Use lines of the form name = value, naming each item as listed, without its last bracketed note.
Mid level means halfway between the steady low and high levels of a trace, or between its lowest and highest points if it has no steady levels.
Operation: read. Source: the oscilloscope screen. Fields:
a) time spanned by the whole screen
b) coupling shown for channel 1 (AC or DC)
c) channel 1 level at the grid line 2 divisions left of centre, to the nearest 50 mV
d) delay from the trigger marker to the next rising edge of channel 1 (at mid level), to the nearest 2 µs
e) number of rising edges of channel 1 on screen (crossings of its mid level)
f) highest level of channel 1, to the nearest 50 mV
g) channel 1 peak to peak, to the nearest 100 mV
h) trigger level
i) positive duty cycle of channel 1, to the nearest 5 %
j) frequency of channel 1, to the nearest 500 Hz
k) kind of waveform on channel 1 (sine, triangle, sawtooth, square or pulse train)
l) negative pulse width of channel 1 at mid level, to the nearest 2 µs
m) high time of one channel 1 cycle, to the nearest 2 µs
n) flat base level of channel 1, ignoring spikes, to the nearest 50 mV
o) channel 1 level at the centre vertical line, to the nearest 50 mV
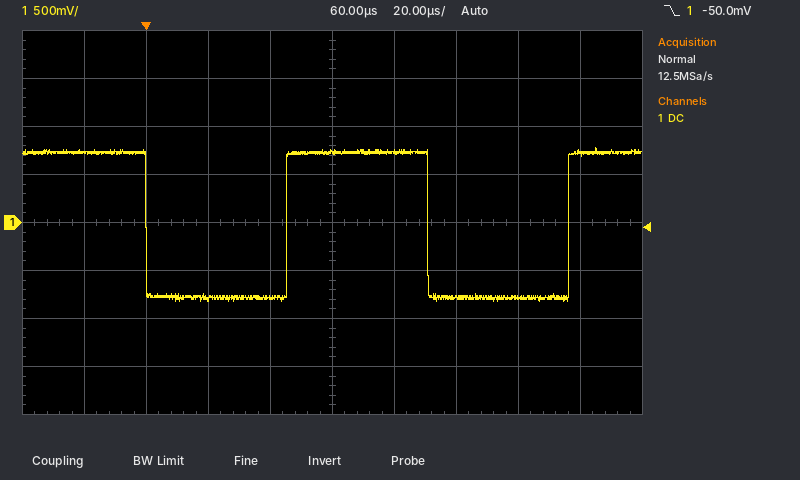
time spanned by the whole screen = 200 µs
coupling shown for channel 1 = DC
channel 1 level at the grid line 2 divisions left of centre, to the nearest 50 mV = -800 mV
delay from the trigger marker to the next rising edge of channel 1 (at mid level), to the nearest 2 µs = 46 µs
number of rising edges of channel 1 on screen = 2
highest level of channel 1, to the nearest 50 mV = 800 mV
channel 1 peak to peak, to the nearest 100 mV = 1.60 V
trigger level = -50.0 mV
positive duty cycle of channel 1, to the nearest 5 % = 50 %
frequency of channel 1, to the nearest 500 Hz = 11.0 kHz
kind of waveform on channel 1 = square
negative pulse width of channel 1 at mid level, to the nearest 2 µs = 46 µs
high time of one channel 1 cycle, to the nearest 2 µs = 46 µs
flat base level of channel 1, ignoring spikes, to the nearest 50 mV = -800 mV
channel 1 level at the centre vertical line, to the nearest 50 mV = 750 mV
